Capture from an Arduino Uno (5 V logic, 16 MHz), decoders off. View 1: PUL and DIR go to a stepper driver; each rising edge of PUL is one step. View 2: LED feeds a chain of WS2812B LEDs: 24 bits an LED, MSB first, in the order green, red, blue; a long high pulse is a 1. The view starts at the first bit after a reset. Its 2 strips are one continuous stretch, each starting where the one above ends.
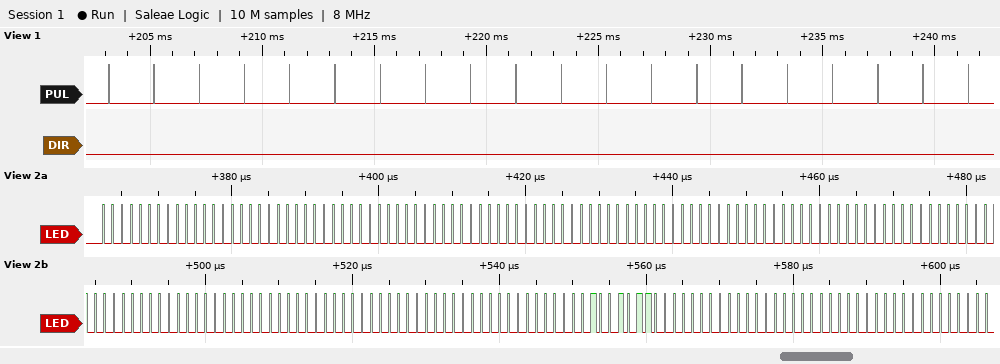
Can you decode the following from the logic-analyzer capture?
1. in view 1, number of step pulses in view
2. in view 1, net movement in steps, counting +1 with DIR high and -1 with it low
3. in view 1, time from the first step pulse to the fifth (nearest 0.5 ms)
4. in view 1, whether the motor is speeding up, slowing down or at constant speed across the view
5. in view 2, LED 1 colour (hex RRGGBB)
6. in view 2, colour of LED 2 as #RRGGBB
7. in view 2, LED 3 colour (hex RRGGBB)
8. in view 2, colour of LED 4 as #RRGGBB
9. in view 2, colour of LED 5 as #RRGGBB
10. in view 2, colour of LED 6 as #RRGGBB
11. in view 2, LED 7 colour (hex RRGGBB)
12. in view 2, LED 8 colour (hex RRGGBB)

20
-20
8.0 ms
constant speed
#000000
#000000
#000000
#000000
#000000
#000000
#960000
#000000
